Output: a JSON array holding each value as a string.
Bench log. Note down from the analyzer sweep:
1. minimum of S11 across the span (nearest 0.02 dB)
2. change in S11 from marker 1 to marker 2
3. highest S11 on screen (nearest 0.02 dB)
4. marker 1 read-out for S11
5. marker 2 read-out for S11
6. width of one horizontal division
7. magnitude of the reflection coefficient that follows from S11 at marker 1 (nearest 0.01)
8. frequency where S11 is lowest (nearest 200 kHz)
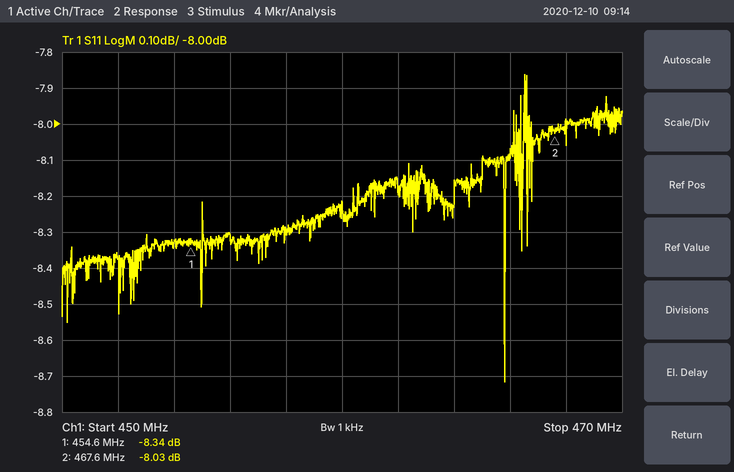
["-8.72 dB", "0.31 dB", "-7.86 dB", "-8.34 dB", "-8.03 dB", "2 MHz", "0.38", "465.8 MHz"]
